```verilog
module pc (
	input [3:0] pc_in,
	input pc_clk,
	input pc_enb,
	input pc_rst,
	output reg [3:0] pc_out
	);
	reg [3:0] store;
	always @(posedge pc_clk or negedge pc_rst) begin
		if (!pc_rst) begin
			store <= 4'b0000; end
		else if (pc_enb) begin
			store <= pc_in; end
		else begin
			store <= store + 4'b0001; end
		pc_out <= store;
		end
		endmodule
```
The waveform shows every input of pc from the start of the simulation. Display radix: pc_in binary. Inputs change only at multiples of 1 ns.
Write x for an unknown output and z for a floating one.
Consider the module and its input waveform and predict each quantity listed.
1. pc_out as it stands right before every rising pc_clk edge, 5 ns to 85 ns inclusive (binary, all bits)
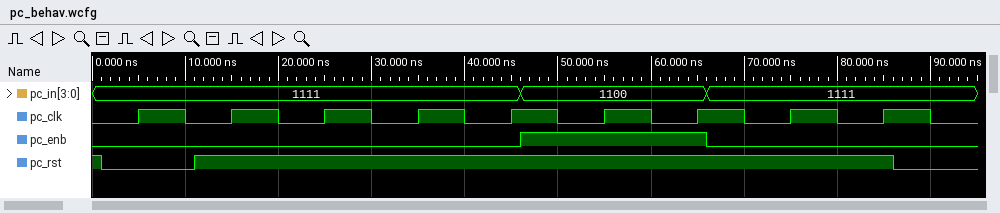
x, 0000, 0000, 0001, 0010, 0011, 0100, 1100, 1100
